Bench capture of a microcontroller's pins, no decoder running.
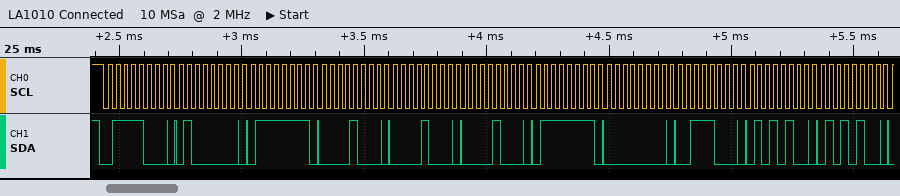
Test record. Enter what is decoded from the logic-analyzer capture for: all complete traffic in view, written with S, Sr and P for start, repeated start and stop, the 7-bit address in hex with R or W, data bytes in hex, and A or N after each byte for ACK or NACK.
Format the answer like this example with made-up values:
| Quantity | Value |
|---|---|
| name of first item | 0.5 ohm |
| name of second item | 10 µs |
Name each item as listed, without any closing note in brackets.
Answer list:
| Quantity | Value |
|---|---|
| all complete traffic in view, written with S, Sr and P for start, repeated start and stop, the 7-bit address in hex with R or W, data bytes in hex, and A or N after each byte for ACK or NACK | S 3CW A 40 A 7F A 08 A 08 A 08 A 7F A 00 A 38 A 54 A 54 A |
